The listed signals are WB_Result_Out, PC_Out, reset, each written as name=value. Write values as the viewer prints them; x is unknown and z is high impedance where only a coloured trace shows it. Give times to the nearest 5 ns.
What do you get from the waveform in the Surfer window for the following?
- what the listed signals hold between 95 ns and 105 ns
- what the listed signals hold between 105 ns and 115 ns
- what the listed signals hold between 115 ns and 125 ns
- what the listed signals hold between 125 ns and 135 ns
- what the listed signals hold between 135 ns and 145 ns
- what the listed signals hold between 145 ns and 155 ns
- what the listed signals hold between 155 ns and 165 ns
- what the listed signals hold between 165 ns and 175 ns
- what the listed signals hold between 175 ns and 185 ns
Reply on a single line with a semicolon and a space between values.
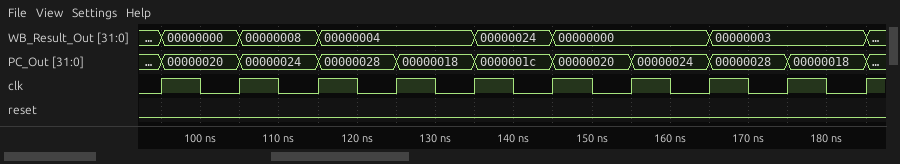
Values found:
WB_Result_Out=00000000, PC_Out=00000020, reset=0; WB_Result_Out=00000008, PC_Out=00000024, reset=0; WB_Result_Out=00000004, PC_Out=00000028, reset=0; WB_Result_Out=00000004, PC_Out=00000018, reset=0; WB_Result_Out=00000024, PC_Out=0000001c, reset=0; WB_Result_Out=00000000, PC_Out=00000020, reset=0; WB_Result_Out=00000000, PC_Out=00000024, reset=0; WB_Result_Out=00000003, PC_Out=00000028, reset=0; WB_Result_Out=00000003, PC_Out=00000018, reset=0
